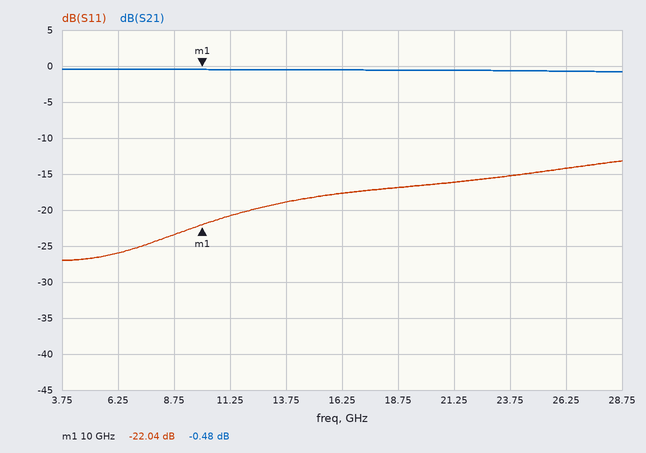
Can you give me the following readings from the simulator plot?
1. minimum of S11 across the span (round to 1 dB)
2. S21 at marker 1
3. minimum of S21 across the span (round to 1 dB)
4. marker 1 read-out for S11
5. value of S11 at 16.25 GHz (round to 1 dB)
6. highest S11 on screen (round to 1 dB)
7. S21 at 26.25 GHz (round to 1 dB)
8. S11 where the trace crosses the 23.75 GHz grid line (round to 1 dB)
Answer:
-27 dB
-0.48 dB
-1 dB
-22.04 dB
-18 dB
-13 dB
-1 dB
-15 dB
